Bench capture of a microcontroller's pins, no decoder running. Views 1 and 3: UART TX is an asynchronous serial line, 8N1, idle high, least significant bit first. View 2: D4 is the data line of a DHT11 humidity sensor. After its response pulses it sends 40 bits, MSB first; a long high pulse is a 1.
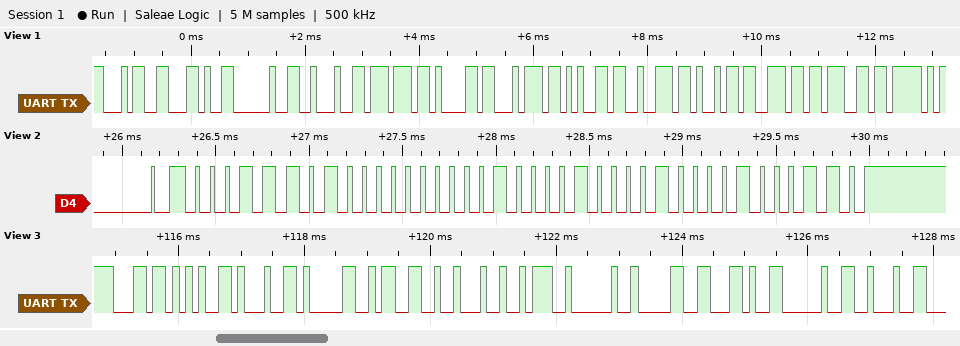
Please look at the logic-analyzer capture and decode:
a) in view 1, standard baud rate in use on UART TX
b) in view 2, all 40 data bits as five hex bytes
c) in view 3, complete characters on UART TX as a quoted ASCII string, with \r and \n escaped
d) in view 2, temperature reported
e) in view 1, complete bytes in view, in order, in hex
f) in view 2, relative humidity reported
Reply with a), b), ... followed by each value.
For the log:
a) 9600 baud
b) 1D 00 21 08 46
c) "led03\": 0, \""
d) 33.8 °C
e) 34 2C 20 22 77 61 74 65 72 69 6E 67 5F
f) 29 %
